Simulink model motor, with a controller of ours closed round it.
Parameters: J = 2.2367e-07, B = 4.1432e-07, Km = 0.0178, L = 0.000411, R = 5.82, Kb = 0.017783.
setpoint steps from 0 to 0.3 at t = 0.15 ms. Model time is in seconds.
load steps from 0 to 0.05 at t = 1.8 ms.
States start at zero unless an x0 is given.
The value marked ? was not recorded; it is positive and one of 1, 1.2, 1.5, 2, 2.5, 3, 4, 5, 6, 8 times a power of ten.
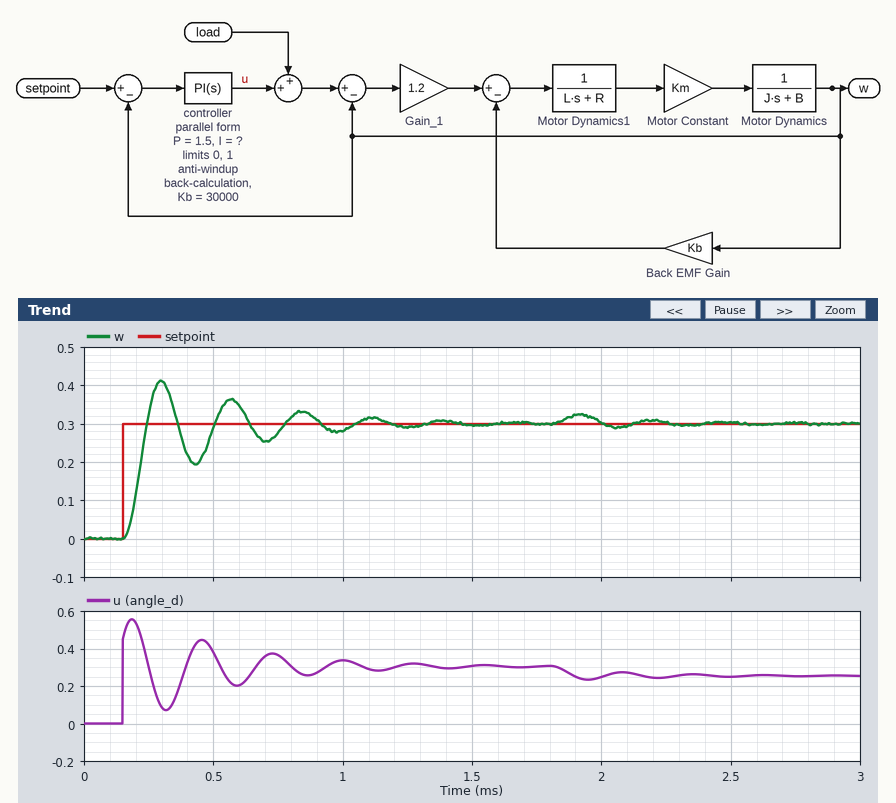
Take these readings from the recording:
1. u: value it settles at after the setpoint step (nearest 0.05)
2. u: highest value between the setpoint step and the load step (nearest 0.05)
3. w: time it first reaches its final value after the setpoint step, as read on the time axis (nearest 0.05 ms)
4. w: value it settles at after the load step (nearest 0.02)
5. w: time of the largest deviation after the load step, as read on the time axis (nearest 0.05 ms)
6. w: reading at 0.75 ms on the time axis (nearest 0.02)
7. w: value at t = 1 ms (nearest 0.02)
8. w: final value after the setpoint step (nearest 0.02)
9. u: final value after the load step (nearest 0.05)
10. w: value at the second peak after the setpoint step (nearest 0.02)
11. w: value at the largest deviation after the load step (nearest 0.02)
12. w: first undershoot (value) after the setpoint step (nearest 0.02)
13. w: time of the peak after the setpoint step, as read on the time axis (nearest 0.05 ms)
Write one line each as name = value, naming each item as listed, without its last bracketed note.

u: value it settles at after the setpoint step = 0.30
u: highest value between the setpoint step and the load step = 0.55
w: time it first reaches its final value after the setpoint step, as read on the time axis = 0.25 ms
w: value it settles at after the load step = 0.30
w: time of the largest deviation after the load step, as read on the time axis = 1.90 ms
w: reading at 0.75 ms on the time axis = 0.28
w: value at t = 1 ms = 0.28
w: final value after the setpoint step = 0.30
u: final value after the load step = 0.25
w: value at the second peak after the setpoint step = 0.36
w: value at the largest deviation after the load step = 0.32
w: first undershoot (value) after the setpoint step = 0.20
w: time of the peak after the setpoint step, as read on the time axis = 0.30 ms
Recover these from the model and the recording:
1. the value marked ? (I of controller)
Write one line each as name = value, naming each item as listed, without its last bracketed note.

the value marked ? = 20000
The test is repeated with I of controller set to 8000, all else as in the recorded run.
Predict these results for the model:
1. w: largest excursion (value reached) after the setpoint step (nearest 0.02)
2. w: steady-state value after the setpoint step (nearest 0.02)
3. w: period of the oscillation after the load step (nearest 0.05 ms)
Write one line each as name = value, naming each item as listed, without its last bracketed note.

w: largest excursion (value reached) after the setpoint step = 0.32
w: steady-state value after the setpoint step = 0.30
w: period of the oscillation after the load step = 0.25 ms
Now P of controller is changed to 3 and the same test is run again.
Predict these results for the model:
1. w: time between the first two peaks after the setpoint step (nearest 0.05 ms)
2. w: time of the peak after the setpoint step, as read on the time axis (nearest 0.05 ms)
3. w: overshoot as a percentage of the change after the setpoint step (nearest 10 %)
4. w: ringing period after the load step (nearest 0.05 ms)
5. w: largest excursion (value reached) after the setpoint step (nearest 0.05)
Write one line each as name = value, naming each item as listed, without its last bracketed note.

w: time between the first two peaks after the setpoint step = 0.20 ms
w: time of the peak after the setpoint step, as read on the time axis = 0.25 ms
w: overshoot as a percentage of the change after the setpoint step = 40 %
w: ringing period after the load step = 0.20 ms
w: largest excursion (value reached) after the setpoint step = 0.40
